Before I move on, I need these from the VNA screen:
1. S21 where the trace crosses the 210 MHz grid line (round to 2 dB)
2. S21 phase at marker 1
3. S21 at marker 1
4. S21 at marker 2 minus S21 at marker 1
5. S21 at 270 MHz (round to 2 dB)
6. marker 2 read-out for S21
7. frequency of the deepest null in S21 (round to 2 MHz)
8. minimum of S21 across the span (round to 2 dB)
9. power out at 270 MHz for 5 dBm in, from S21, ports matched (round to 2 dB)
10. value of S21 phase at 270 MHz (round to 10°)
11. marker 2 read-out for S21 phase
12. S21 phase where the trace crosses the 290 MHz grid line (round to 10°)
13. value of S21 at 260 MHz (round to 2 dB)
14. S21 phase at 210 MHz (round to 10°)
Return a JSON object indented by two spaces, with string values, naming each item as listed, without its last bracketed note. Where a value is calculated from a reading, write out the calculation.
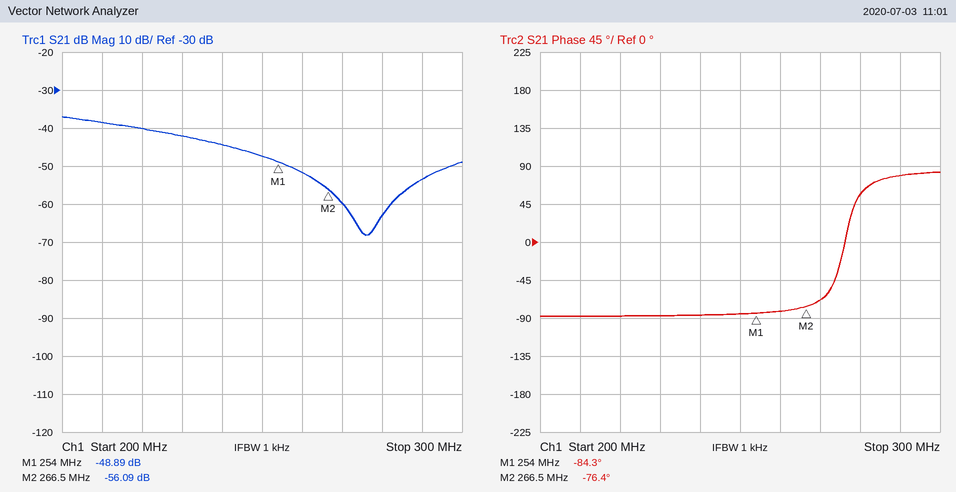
{
  "S21 where the trace crosses the 210 MHz grid line": "-38 dB",
  "S21 phase at marker 1": "-84.3°",
  "S21 at marker 1": "-48.89 dB",
  "S21 at marker 2 minus S21 at marker 1": "-56.09 − (-48.89) = -7.20 dB",
  "S21 at 270 MHz": "-60 dB",
  "marker 2 read-out for S21": "-56.09 dB",
  "frequency of the deepest null in S21": "276 MHz",
  "minimum of S21 across the span": "-68 dB",
  "power out at 270 MHz for 5 dBm in, from S21, ports matched": "5 dBm + (-60 dB) = -54 dBm",
  "value of S21 phase at 270 MHz": "-70°",
  "marker 2 read-out for S21 phase": "-76.4°",
  "S21 phase where the trace crosses the 290 MHz grid line": "80°",
  "value of S21 at 260 MHz": "-52 dB",
  "S21 phase at 210 MHz": "-90°"
}
